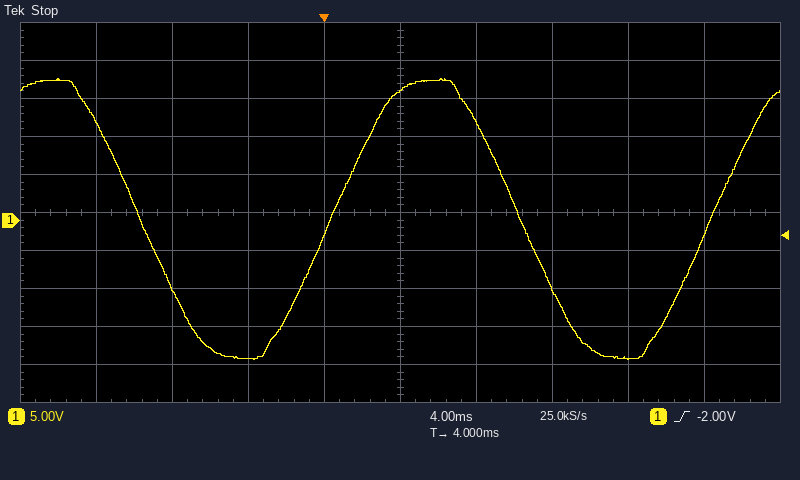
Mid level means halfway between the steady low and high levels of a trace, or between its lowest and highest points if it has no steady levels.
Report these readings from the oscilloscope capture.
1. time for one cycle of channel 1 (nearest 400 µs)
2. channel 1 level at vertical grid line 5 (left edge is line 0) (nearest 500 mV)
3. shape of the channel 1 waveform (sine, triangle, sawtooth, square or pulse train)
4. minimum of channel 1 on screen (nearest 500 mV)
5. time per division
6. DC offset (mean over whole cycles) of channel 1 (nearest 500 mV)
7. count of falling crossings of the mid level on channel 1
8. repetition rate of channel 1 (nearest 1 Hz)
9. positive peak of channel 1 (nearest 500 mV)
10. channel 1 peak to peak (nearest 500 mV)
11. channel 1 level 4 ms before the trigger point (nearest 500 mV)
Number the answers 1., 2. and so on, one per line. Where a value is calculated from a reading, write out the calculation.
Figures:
1. 20.0 ms
2. 17.0 V
3. sine
4. -18.5 V
5. 4 ms
6. (18.5 V + (-18.5 V)) / 2 ≈ 0.0 V
7. 2
8. 1 / 20.0 ms ≈ 50 Hz
9. 18.5 V
10. 18.5 V − (-18.5 V) = 37.0 V
11. -18.0 V
